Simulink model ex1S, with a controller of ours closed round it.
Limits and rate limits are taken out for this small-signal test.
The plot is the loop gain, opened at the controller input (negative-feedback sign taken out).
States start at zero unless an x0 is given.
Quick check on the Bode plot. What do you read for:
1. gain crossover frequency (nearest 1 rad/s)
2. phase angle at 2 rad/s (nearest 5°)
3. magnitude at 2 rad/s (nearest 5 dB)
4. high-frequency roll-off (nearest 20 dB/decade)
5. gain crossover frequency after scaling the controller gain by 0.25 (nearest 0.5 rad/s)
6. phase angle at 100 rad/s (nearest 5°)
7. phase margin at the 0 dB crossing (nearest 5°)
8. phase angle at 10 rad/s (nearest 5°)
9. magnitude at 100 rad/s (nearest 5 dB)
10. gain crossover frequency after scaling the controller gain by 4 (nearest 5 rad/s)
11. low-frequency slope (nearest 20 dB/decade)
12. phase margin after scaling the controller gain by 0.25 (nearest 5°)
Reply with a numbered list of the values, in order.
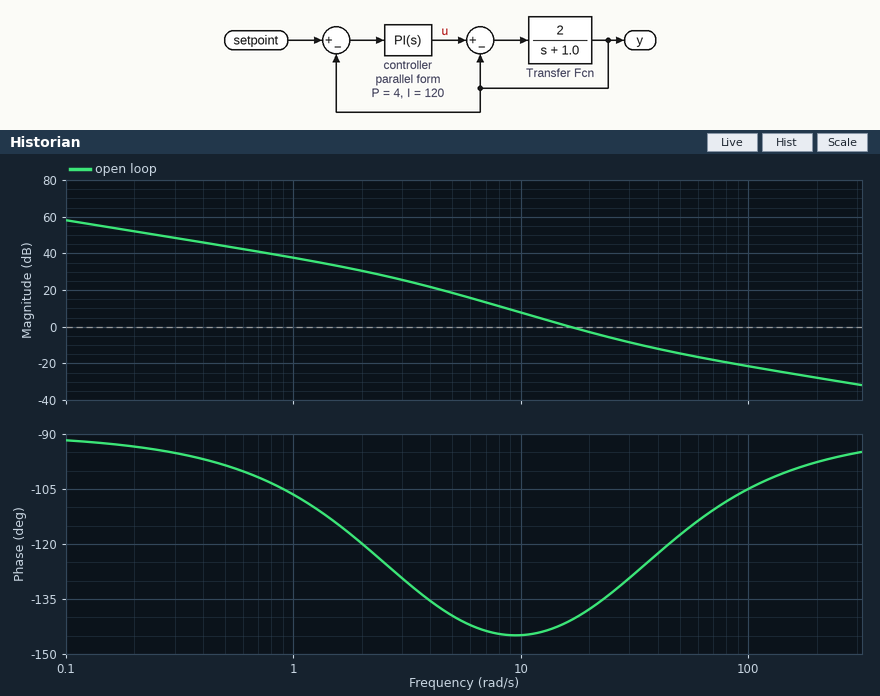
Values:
1. 16 rad/s
2. -120°
3. 30 dB
4. -20 dB/decade
5. 7.5 rad/s
6. -105°
7. 40°
8. -145°
9. -20 dB
10. 40 rad/s
11. -20 dB/decade
12. 35°
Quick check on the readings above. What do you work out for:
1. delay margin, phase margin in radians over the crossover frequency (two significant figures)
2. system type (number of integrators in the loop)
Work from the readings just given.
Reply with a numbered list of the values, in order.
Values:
1. 0.044 s
2. 1
